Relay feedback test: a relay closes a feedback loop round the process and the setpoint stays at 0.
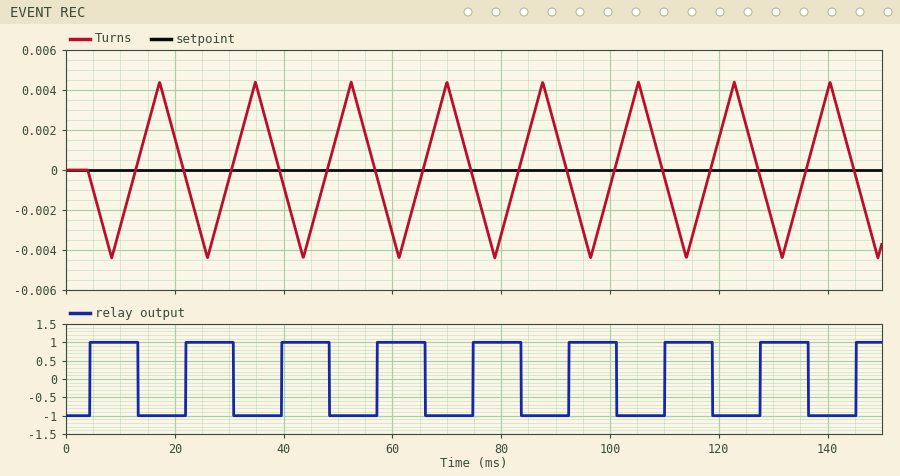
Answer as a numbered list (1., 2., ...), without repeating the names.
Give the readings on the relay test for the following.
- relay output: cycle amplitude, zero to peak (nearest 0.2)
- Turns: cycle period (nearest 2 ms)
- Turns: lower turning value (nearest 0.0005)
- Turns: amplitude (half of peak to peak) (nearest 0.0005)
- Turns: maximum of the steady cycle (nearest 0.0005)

1. 1.0
2. 18 ms
3. -0.0045
4. 0.0045
5. 0.0045
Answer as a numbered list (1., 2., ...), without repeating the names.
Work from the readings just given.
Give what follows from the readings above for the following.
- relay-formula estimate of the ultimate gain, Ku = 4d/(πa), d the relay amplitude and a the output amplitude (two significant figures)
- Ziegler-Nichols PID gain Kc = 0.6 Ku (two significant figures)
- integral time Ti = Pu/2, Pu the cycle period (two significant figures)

1. 280
2. 170
3. 9.0 ms
